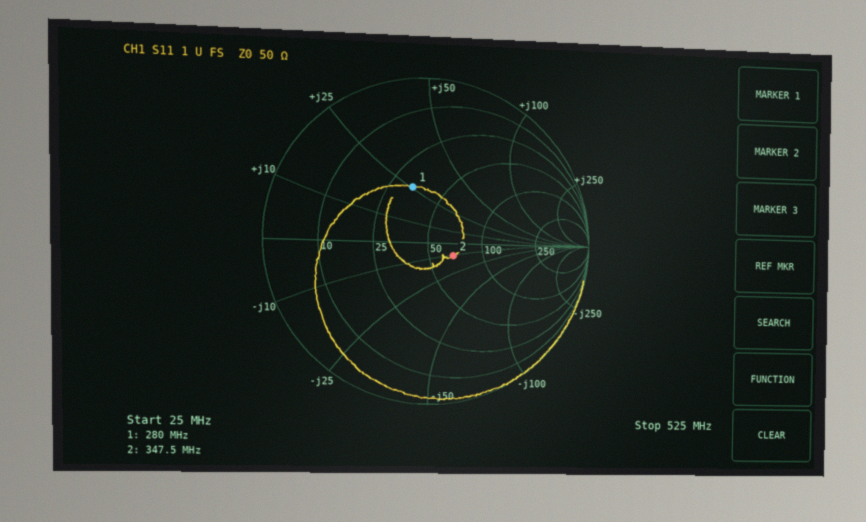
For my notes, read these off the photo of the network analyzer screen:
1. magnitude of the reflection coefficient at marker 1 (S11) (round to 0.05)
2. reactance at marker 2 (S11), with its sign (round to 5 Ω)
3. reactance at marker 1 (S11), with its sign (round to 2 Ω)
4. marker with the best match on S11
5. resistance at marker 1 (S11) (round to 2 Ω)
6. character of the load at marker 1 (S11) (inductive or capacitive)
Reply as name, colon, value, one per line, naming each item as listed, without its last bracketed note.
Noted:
magnitude of the reflection coefficient at marker 1 (S11): 0.35
reactance at marker 2 (S11), with its sign: -10 Ω
reactance at marker 1 (S11), with its sign: +26 Ω
marker with the best match on S11: marker 2
resistance at marker 1 (S11): 34 Ω
character of the load at marker 1 (S11): inductive
